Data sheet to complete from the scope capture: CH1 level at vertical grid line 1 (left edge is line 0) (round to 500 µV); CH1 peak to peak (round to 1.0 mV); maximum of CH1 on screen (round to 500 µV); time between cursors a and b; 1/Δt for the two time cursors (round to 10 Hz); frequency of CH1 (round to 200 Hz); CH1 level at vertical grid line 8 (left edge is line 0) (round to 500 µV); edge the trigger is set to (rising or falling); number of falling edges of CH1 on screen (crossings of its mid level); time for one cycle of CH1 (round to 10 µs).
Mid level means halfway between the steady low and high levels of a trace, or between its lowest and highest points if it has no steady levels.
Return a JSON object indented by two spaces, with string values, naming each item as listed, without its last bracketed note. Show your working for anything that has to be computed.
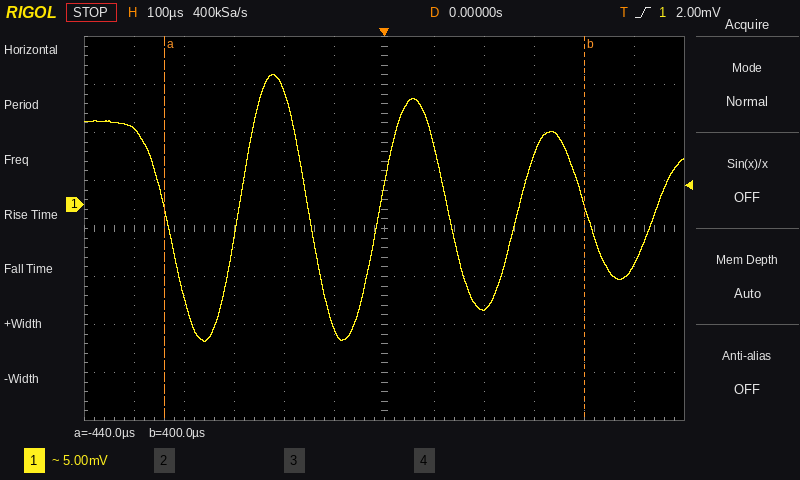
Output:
{
  "CH1 level at vertical grid line 1 (left edge is line 0)": "8.0 mV",
  "CH1 peak to peak": "28.0 mV",
  "maximum of CH1 on screen": "13.5 mV",
  "time between cursors a and b": "400 µs − (-440 µs) = 840 µs",
  "1/Δt for the two time cursors": "1 / 840 µs ≈ 1.19 kHz",
  "frequency of CH1": "1 / 280 µs ≈ 3.6 kHz",
  "CH1 level at vertical grid line 8 (left edge is line 0)": "-11.0 mV",
  "edge the trigger is set to": "rising",
  "number of falling edges of CH1 on screen": "4",
  "time for one cycle of CH1": "280 µs"
}
